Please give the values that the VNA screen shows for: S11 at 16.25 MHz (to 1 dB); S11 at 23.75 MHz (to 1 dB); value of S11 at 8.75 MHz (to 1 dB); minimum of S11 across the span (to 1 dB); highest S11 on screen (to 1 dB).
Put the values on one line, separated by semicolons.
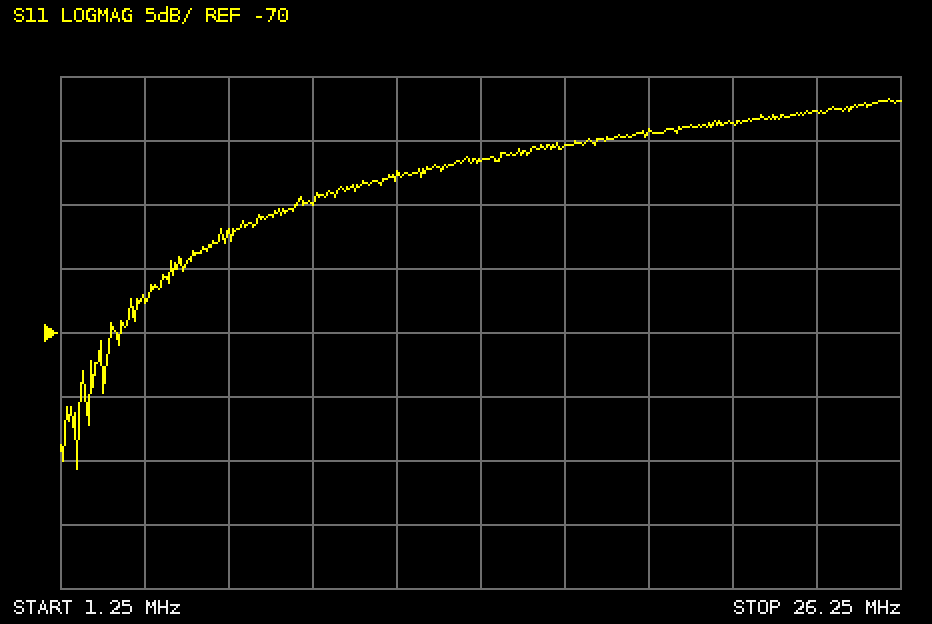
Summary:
-55 dB; -53 dB; -60 dB; -81 dB; -52 dB
